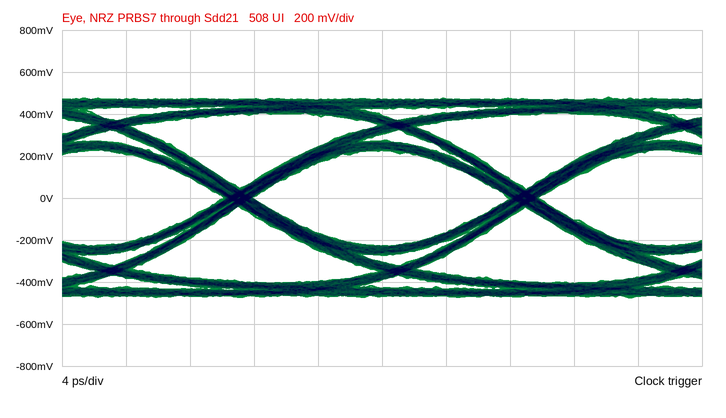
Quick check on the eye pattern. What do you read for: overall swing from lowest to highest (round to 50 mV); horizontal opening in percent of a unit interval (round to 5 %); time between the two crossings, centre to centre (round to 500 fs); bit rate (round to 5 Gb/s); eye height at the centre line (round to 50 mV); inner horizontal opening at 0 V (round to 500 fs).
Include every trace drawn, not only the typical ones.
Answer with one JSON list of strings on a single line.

["950 mV", "90 %", "18.0 ps", "55 Gb/s", "450 mV", "16.0 ps"]
